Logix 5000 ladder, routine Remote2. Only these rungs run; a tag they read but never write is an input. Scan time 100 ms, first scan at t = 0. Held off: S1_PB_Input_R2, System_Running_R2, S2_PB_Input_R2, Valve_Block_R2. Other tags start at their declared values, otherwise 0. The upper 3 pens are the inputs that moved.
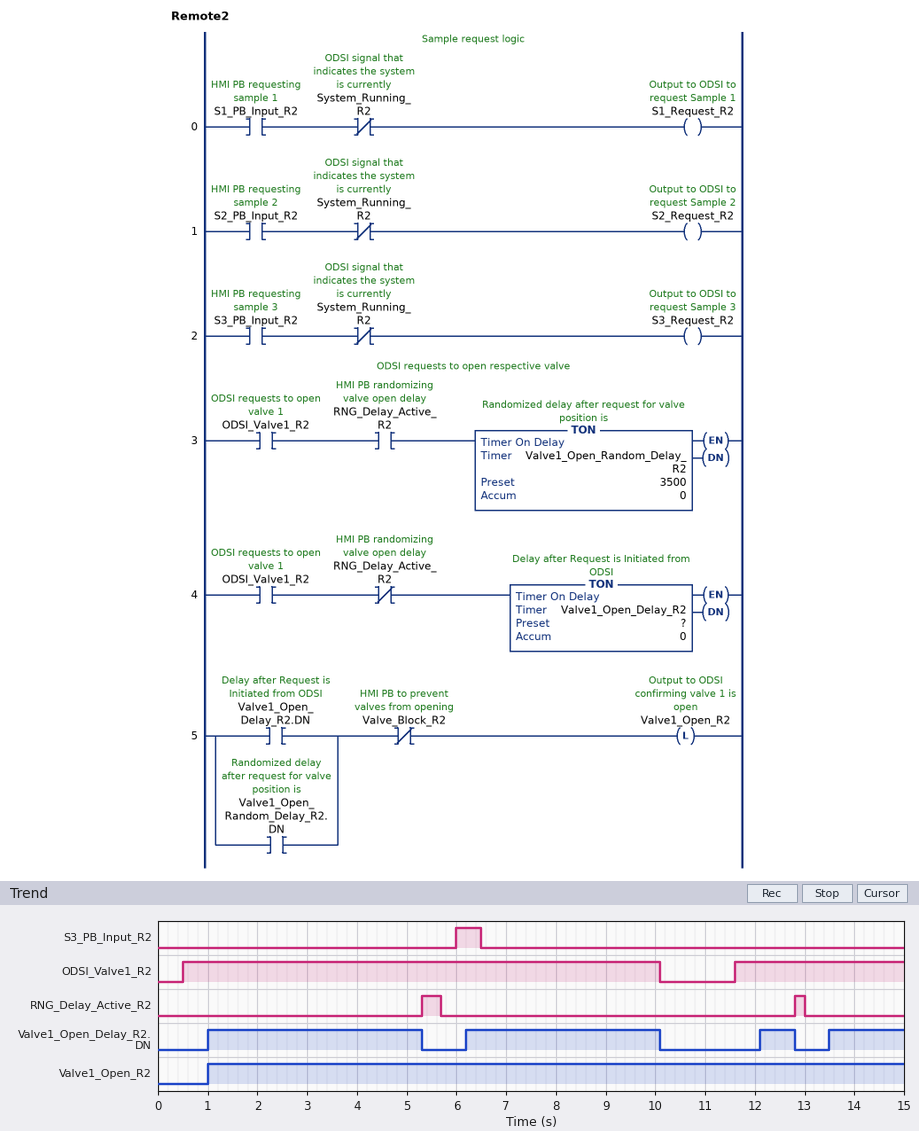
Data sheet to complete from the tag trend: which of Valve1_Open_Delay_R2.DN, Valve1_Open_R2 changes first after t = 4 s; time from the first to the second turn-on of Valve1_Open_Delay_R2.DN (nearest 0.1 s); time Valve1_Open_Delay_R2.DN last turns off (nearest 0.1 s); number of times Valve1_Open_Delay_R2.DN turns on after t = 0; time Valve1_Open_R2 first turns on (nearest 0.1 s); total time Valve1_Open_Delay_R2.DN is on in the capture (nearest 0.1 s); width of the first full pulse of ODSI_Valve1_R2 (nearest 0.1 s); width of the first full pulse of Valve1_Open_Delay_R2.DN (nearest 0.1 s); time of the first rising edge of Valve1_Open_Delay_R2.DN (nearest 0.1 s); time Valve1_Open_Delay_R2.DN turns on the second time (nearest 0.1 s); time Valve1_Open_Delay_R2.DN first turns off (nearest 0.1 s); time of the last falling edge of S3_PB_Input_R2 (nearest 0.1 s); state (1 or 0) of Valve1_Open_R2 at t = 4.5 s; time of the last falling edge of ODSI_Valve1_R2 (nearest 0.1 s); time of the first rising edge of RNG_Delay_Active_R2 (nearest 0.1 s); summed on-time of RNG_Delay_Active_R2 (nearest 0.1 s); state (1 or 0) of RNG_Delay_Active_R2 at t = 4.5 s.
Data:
Valve1_Open_Delay_R2.DN
5.2 s
12.8 s
4
1.0 s
10.4 s
9.6 s
4.3 s
1.0 s
6.2 s
5.3 s
6.5 s
1
10.1 s
5.3 s
0.6 s
0
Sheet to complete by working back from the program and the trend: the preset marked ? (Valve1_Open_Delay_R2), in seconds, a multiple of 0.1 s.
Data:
0.5 s
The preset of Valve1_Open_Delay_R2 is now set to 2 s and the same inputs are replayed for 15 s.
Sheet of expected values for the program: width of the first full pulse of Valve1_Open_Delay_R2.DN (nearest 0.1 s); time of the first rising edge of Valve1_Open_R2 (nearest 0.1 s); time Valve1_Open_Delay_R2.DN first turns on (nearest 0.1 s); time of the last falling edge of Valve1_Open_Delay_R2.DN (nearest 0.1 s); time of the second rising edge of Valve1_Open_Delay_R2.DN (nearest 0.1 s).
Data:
2.8 s
2.5 s
2.5 s
10.1 s
7.7 s
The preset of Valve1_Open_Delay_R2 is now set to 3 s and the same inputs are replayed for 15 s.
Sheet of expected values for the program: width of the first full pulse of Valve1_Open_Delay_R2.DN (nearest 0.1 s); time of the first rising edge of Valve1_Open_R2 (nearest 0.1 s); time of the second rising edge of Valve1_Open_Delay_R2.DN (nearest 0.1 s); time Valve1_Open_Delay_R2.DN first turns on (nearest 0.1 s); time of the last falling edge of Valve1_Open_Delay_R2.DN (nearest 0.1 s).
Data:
1.8 s
3.5 s
8.7 s
3.5 s
10.1 s
